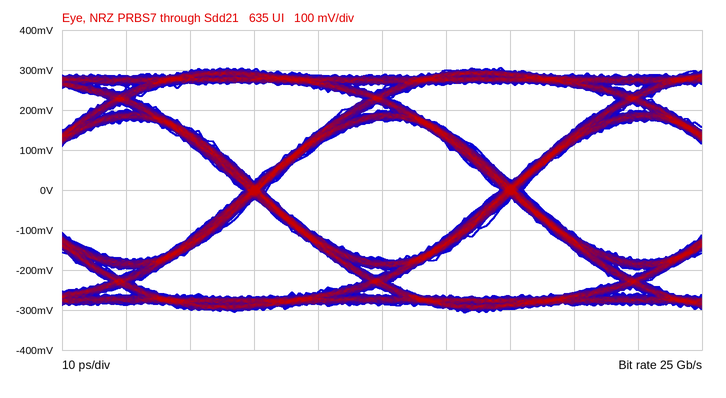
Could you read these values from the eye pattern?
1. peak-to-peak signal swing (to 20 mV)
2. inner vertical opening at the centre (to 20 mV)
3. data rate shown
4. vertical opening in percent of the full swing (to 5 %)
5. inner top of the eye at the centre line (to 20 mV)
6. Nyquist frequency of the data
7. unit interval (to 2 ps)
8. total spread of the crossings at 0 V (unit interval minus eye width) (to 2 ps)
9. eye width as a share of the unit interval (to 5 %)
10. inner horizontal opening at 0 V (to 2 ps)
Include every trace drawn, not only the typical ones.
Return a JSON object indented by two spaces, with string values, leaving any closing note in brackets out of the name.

{
  "peak-to-peak signal swing": "620 mV",
  "inner vertical opening at the centre": "340 mV",
  "data rate shown": "25 Gb/s",
  "vertical opening in percent of the full swing": "55 %",
  "inner top of the eye at the centre line": "180 mV",
  "Nyquist frequency of the data": "12.5 GHz",
  "unit interval": "40 ps",
  "total spread of the crossings at 0 V (unit interval minus eye width)": "4 ps",
  "eye width as a share of the unit interval": "90 %",
  "inner horizontal opening at 0 V": "36 ps"
}
